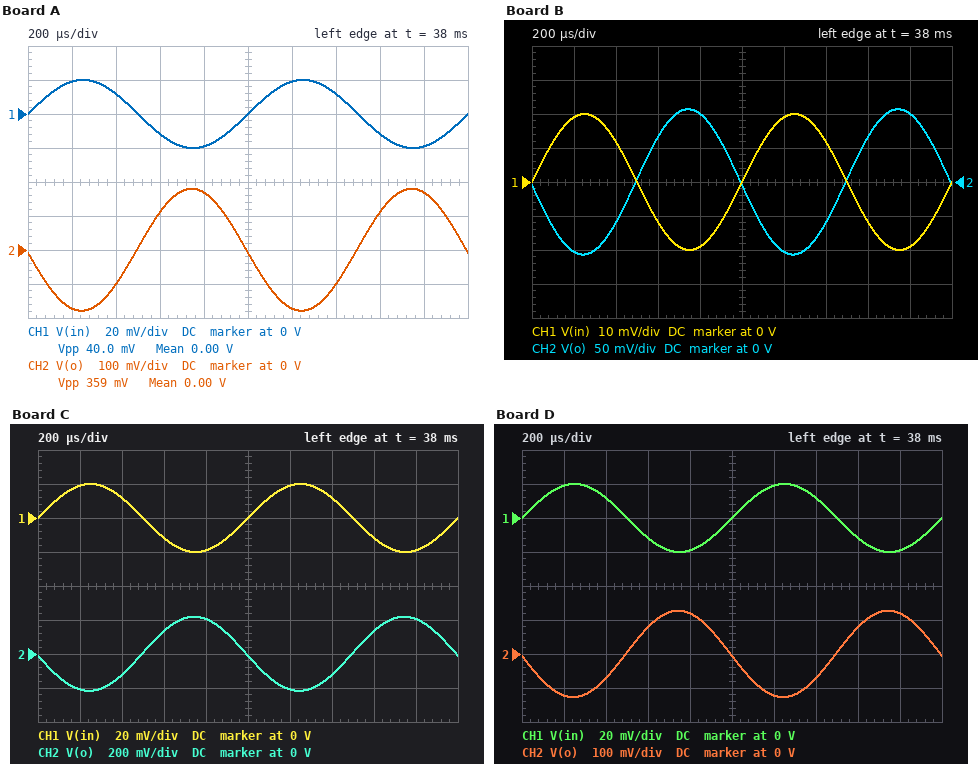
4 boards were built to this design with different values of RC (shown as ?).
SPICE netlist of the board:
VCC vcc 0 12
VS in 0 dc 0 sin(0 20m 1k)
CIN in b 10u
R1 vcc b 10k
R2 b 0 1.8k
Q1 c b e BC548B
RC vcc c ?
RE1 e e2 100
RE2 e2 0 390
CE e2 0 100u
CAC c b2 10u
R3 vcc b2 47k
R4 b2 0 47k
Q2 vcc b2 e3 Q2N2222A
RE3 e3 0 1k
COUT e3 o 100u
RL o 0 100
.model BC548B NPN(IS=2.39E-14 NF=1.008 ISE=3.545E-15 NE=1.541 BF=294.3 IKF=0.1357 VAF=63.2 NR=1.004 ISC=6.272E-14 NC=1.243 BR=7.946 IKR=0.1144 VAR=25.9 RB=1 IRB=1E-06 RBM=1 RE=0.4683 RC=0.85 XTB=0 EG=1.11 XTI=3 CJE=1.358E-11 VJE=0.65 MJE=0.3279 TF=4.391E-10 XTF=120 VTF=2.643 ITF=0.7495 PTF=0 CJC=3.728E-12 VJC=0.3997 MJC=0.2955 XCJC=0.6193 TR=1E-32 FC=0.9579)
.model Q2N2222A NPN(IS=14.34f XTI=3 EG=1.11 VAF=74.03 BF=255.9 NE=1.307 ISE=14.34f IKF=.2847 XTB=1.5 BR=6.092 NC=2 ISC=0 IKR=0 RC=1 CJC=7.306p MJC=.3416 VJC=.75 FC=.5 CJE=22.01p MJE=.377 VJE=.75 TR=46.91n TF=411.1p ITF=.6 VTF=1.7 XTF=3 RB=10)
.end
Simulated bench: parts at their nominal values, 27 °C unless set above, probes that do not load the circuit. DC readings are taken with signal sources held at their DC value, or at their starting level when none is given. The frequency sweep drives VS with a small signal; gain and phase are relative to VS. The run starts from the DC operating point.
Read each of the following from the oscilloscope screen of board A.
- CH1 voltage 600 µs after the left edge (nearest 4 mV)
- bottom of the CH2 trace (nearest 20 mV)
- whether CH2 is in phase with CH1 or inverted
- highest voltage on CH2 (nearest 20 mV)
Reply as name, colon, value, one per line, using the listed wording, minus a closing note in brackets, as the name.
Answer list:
CH1 voltage 600 µs after the left edge: -12 mV
bottom of the CH2 trace: -180 mV
whether CH2 is in phase with CH1 or inverted: inverted
highest voltage on CH2: 180 mV
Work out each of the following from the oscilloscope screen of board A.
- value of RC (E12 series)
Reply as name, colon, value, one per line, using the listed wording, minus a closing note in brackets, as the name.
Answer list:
value of RC: 1.2 kΩ
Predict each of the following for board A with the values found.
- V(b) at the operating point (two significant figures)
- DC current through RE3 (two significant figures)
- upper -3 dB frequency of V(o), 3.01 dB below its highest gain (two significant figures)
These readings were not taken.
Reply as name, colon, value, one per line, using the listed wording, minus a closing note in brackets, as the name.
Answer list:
V(b) at the operating point: 1.8 V
DC current through RE3: 4.7 mA
upper -3 dB frequency of V(o), 3.01 dB below its highest gain: 13 MHz
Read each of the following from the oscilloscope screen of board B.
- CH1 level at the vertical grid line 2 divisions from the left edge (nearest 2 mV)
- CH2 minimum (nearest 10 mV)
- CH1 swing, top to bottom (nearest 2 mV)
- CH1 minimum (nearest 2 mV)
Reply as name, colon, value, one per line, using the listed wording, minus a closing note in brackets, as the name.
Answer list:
CH1 level at the vertical grid line 2 divisions from the left edge: 12 mV
CH2 minimum: -110 mV
CH1 swing, top to bottom: 40 mV
CH1 minimum: -20 mV
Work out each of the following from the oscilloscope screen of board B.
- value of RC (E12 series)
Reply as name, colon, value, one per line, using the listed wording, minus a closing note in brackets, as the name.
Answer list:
value of RC: 680 Ω
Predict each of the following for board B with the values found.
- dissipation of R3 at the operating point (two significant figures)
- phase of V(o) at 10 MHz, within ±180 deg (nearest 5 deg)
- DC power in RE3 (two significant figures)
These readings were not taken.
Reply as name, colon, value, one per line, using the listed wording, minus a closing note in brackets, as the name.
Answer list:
dissipation of R3 at the operating point: 930 µW
phase of V(o) at 10 MHz, within ±180 deg: 150 deg
DC power in RE3: 22 mW
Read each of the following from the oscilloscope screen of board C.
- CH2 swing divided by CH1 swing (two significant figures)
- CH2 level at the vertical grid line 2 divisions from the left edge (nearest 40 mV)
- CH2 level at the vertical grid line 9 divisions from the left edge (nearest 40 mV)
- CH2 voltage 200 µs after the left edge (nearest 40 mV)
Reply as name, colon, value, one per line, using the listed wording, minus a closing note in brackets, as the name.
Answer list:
CH2 swing divided by CH1 swing: 11
CH2 level at the vertical grid line 2 divisions from the left edge: -120 mV
CH2 level at the vertical grid line 9 divisions from the left edge: 200 mV
CH2 voltage 200 µs after the left edge: -200 mV
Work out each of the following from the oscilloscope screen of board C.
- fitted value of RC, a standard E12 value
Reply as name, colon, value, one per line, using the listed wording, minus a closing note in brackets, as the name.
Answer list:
fitted value of RC, a standard E12 value: 1.5 kΩ
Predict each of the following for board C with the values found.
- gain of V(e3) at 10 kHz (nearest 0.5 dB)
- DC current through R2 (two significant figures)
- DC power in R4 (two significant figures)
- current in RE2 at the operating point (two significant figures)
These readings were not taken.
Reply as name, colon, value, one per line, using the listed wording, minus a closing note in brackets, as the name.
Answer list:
gain of V(e3) at 10 kHz: 21.0 dB
DC current through R2: 1.0 mA
DC power in R4: 620 µW
current in RE2 at the operating point: 2.4 mA
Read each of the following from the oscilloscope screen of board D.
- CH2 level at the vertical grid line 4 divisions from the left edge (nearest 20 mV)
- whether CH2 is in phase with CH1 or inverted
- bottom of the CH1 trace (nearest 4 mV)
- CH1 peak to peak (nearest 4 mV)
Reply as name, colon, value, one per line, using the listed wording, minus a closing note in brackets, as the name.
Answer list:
CH2 level at the vertical grid line 4 divisions from the left edge: 120 mV
whether CH2 is in phase with CH1 or inverted: inverted
bottom of the CH1 trace: -20 mV
CH1 peak to peak: 40 mV
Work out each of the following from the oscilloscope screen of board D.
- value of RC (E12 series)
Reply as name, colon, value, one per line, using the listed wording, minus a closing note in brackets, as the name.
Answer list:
value of RC: 820 Ω
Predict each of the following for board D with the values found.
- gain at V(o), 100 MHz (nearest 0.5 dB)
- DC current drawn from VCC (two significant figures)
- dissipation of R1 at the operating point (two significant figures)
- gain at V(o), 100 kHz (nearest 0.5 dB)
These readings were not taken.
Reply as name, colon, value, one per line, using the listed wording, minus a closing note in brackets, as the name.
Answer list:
gain at V(o), 100 MHz: 0.5 dB
DC current drawn from VCC: 8.2 mA
dissipation of R1 at the operating point: 10 mW
gain at V(o), 100 kHz: 16.0 dB
